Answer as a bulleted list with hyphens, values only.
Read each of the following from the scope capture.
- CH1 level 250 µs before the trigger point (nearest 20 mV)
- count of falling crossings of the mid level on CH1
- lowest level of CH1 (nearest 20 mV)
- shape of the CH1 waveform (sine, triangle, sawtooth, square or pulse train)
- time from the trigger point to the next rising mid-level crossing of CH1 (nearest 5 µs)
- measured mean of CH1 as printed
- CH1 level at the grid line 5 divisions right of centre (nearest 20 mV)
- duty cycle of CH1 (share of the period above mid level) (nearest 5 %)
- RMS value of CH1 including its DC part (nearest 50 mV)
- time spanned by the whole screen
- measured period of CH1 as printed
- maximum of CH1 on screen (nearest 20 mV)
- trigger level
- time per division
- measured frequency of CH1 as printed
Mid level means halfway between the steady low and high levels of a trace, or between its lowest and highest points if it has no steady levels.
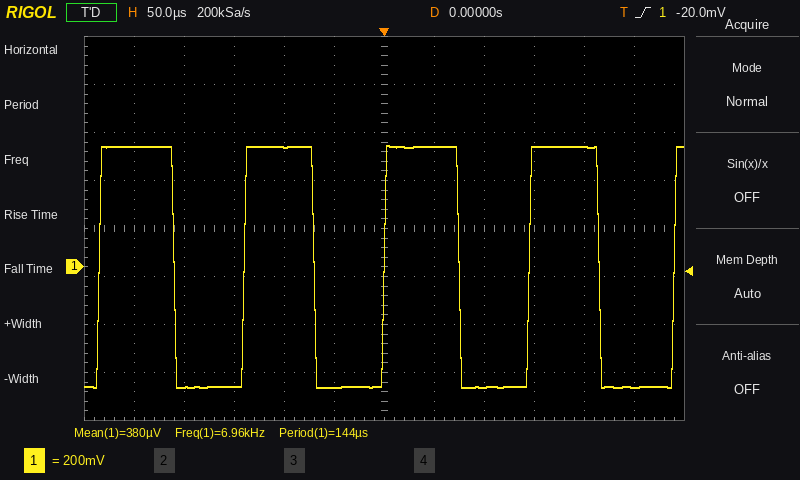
- 500 mV
- 4
- -500 mV
- square
- 145 µs
- 380 µV
- -500 mV
- 50 %
- 500 mV
- 600 µs
- 144 µs
- 500 mV
- -20.0 mV
- 50 µs
- 6.96 kHz
